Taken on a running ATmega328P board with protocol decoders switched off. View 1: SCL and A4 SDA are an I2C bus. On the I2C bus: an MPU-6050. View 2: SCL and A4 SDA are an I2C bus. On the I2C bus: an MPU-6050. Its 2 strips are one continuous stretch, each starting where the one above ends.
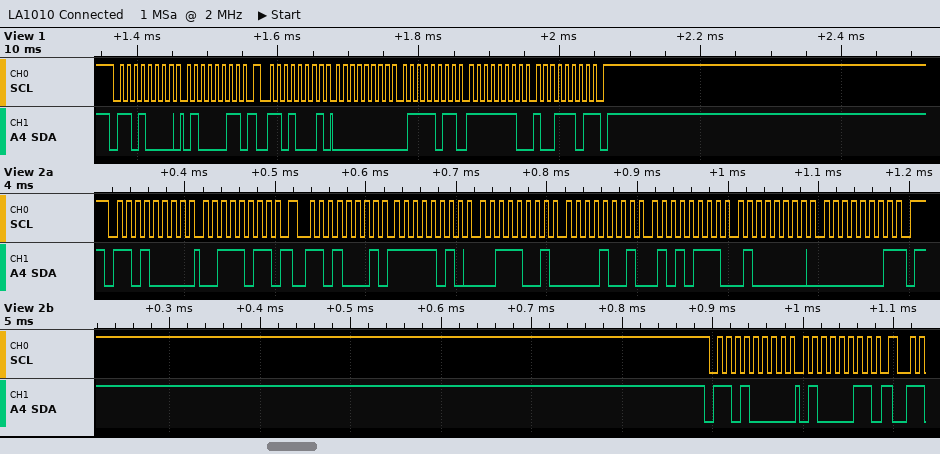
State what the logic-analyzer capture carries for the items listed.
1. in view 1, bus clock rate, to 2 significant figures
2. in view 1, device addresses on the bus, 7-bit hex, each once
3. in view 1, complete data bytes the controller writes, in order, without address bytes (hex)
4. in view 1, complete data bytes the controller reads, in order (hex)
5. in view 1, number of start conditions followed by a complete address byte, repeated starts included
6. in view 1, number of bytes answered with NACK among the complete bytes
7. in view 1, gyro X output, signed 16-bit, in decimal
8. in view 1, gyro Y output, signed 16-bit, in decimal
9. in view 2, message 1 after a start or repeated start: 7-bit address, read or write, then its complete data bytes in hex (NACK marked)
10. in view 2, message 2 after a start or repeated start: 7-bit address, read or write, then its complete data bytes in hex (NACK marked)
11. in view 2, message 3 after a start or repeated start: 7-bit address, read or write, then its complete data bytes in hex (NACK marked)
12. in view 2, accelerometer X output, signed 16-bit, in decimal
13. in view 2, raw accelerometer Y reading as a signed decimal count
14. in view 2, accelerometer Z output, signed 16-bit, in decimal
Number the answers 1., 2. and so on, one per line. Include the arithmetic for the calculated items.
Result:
1. 100 kHz
2. 0x68
3. 43
4. 00 7B FE 9D
5. 2
6. 1
7. 0x007B = 123
8. 0xFE9D = -355
9. 0x68 write: 3B
10. 0x68 read: FA 39 09 57 40 01 NACK
11. 0x68 write: 43
12. 0xFA39 = -1479
13. 0x0957 = 2391
14. 0x4001 = 16385
